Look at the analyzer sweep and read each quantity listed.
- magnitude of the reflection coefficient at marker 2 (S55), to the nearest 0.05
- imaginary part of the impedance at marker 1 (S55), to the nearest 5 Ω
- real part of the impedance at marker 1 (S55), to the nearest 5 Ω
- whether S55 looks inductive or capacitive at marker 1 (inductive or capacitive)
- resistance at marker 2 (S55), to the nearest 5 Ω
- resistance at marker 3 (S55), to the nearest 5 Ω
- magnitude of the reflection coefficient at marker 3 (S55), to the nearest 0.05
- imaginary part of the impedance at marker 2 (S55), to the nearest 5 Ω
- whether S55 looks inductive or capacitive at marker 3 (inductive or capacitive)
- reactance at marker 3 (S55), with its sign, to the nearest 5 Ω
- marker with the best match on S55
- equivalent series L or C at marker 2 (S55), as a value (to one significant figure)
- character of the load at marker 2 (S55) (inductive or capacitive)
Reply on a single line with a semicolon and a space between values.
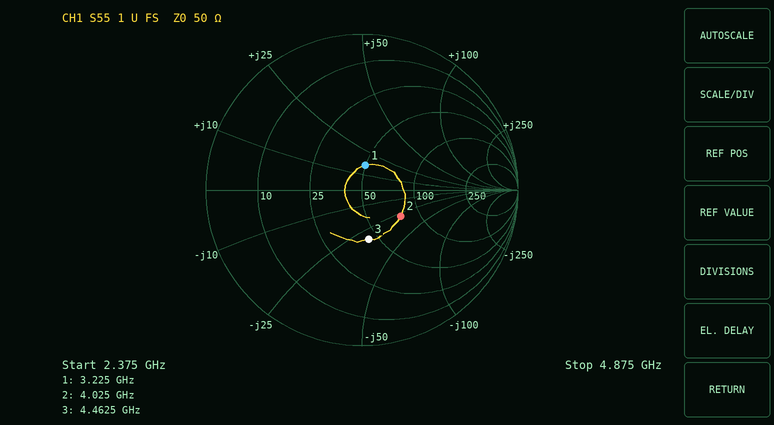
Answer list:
0.30; +15 Ω; 50 Ω; inductive; 75 Ω; 45 Ω; 0.30; -30 Ω; capacitive; -30 Ω; marker 1; 1 pF; capacitive
